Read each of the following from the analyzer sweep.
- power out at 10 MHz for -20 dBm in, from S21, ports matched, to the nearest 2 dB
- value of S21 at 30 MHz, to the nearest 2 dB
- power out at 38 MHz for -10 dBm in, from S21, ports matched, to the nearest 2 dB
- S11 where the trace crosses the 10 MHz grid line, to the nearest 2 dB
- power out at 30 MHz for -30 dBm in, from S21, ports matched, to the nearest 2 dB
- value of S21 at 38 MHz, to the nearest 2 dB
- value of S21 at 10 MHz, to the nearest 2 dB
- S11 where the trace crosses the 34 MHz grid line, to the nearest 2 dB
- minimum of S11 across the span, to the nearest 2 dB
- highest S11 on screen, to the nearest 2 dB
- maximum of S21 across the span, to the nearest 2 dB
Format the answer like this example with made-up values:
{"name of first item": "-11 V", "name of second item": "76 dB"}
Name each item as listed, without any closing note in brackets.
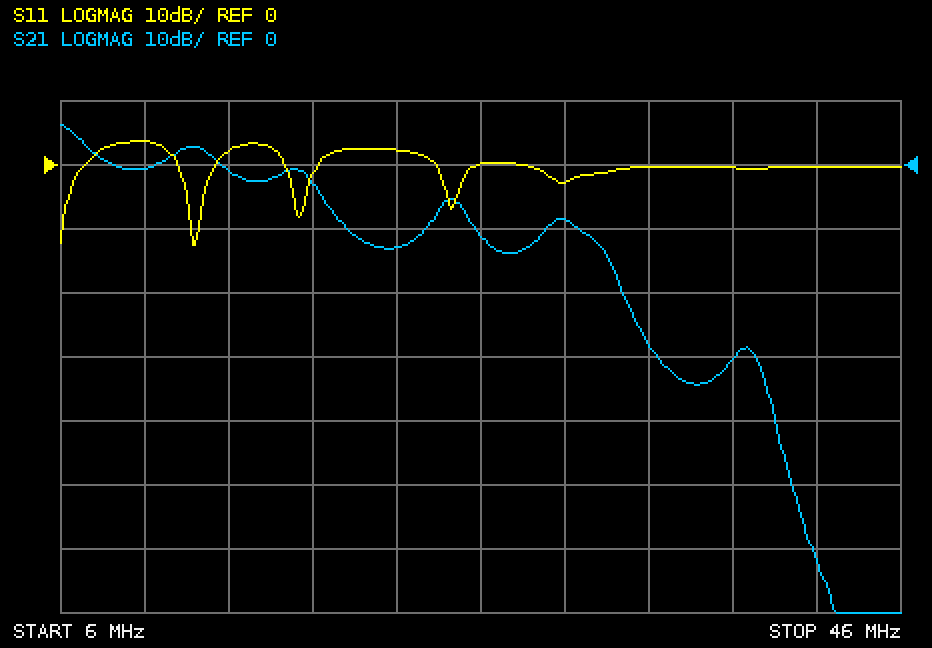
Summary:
{"power out at 10 MHz for -20 dBm in, from S21, ports matched, to the nearest 2 dB": "-20 dBm", "value of S21 at 30 MHz, to the nearest 2 dB": "-8 dB", "power out at 38 MHz for -10 dBm in, from S21, ports matched, to the nearest 2 dB": "-40 dBm", "S11 where the trace crosses the 10 MHz grid line, to the nearest 2 dB": "4 dB", "power out at 30 MHz for -30 dBm in, from S21, ports matched, to the nearest 2 dB": "-38 dBm", "value of S21 at 38 MHz, to the nearest 2 dB": "-30 dB", "value of S21 at 10 MHz, to the nearest 2 dB": "0 dB", "S11 where the trace crosses the 34 MHz grid line, to the nearest 2 dB": "0 dB", "minimum of S11 across the span, to the nearest 2 dB": "-12 dB", "highest S11 on screen, to the nearest 2 dB": "4 dB", "maximum of S21 across the span, to the nearest 2 dB": "6 dB"}
